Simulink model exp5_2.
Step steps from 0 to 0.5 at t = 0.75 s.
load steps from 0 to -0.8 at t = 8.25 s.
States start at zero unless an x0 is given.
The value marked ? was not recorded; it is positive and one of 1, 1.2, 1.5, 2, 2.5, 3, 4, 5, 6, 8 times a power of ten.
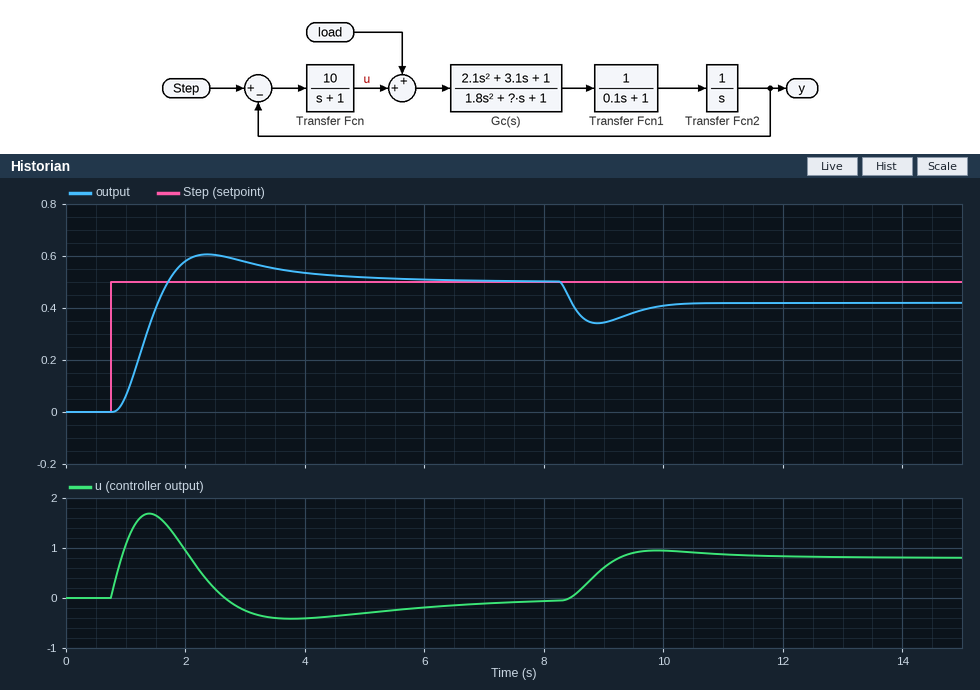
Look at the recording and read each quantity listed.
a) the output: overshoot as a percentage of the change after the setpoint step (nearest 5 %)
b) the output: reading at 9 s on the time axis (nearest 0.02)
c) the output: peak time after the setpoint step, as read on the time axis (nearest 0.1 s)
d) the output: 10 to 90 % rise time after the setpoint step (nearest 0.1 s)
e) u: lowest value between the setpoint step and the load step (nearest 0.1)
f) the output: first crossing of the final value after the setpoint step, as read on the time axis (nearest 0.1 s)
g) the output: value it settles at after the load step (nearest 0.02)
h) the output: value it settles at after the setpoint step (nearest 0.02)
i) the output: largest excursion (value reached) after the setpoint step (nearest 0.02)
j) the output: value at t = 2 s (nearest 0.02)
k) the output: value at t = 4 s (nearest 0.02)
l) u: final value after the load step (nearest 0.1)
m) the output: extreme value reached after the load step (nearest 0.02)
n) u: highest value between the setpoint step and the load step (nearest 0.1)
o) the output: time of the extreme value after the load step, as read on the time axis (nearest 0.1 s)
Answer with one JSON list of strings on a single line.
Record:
["20 %", "0.34", "2.4 s", "0.6 s", "-0.4", "1.7 s", "0.42", "0.50", "0.60", "0.58", "0.54", "0.8", "0.34", "1.7", "8.9 s"]
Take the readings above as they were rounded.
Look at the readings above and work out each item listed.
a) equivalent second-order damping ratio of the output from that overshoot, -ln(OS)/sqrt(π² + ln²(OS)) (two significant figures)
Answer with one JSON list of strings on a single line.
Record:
["0.46"]
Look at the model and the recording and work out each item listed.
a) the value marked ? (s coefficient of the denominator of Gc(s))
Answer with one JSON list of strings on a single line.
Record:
["12"]
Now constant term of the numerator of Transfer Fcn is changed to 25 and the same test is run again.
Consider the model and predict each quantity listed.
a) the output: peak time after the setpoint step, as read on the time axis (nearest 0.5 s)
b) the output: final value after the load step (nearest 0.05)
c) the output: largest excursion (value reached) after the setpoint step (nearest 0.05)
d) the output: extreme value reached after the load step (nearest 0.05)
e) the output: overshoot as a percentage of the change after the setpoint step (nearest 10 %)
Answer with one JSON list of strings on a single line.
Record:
["1.5 s", "0.45", "0.70", "0.40", "40 %"]
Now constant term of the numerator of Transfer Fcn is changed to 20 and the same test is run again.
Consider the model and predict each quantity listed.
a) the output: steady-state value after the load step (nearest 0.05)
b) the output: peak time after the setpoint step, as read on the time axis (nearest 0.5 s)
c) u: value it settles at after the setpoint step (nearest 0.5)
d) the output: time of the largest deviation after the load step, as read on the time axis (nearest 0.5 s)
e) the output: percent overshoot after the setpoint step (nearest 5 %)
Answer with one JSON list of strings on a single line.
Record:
["0.45", "1.5 s", "0.0", "8.5 s", "35 %"]
